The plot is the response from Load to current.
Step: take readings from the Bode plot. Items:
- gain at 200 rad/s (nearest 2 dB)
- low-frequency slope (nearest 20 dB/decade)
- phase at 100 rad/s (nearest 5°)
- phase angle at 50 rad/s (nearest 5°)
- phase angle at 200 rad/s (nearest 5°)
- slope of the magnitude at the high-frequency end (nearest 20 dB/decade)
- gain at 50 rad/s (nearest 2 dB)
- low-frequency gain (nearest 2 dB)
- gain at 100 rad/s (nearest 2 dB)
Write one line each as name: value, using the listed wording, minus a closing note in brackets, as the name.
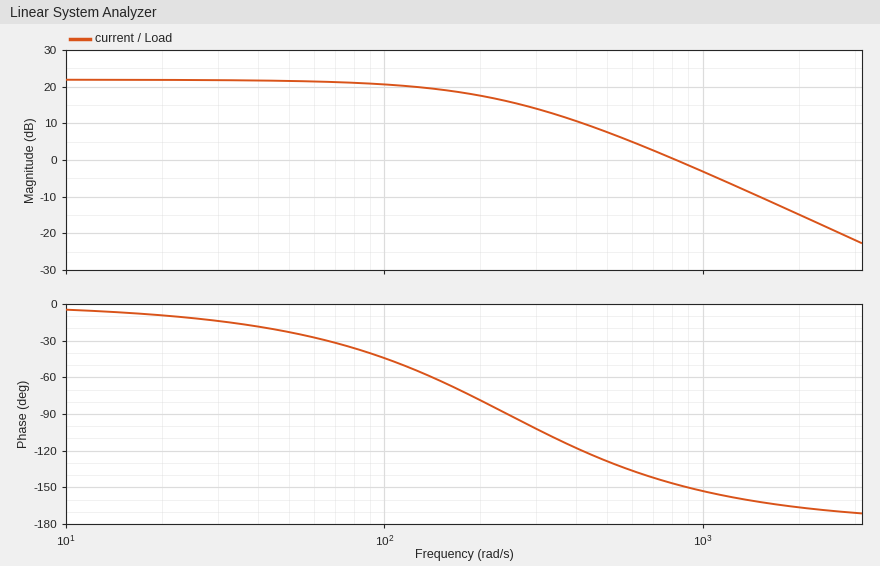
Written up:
gain at 200 rad/s: 18 dB
low-frequency slope: 0 dB/decade
phase at 100 rad/s: -45°
phase angle at 50 rad/s: -25°
phase angle at 200 rad/s: -80°
slope of the magnitude at the high-frequency end: -40 dB/decade
gain at 50 rad/s: 22 dB
low-frequency gain: 22 dB
gain at 100 rad/s: 20 dB
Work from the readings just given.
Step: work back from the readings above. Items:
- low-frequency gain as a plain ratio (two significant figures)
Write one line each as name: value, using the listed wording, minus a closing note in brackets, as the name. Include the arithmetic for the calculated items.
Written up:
low-frequency gain as a plain ratio: 10^(22 / 20) = 13
